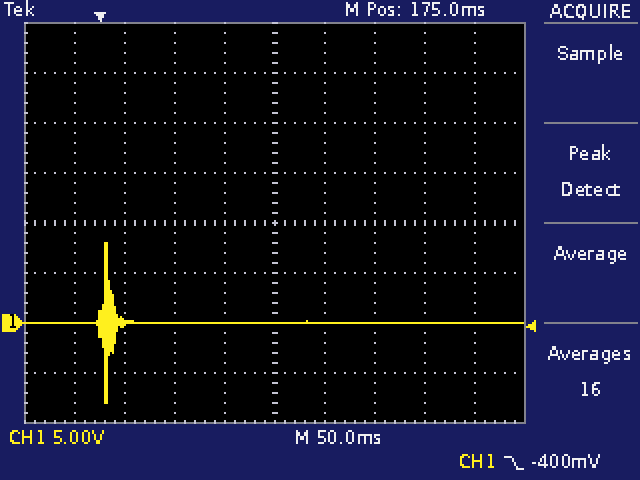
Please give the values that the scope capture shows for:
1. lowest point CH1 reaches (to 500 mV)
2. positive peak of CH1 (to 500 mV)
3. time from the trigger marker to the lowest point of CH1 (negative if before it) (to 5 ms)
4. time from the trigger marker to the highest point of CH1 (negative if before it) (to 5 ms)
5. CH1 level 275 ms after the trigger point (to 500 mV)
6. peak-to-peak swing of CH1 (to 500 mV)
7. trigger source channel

-8.0 V
8.0 V
+5 ms
+5 ms
0.0 V
16.0 V
CH1
